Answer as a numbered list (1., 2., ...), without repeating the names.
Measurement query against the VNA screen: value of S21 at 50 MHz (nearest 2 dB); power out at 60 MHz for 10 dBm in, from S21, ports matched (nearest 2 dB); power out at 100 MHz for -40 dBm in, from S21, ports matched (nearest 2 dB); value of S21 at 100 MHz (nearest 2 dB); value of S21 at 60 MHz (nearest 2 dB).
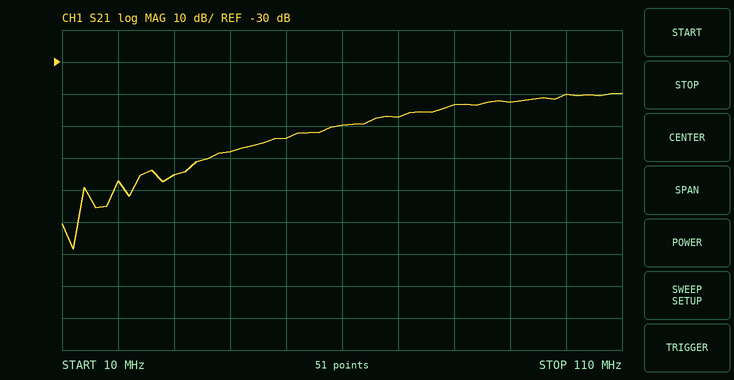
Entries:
1. -54 dB
2. -40 dBm
3. -80 dBm
4. -40 dB
5. -50 dB
